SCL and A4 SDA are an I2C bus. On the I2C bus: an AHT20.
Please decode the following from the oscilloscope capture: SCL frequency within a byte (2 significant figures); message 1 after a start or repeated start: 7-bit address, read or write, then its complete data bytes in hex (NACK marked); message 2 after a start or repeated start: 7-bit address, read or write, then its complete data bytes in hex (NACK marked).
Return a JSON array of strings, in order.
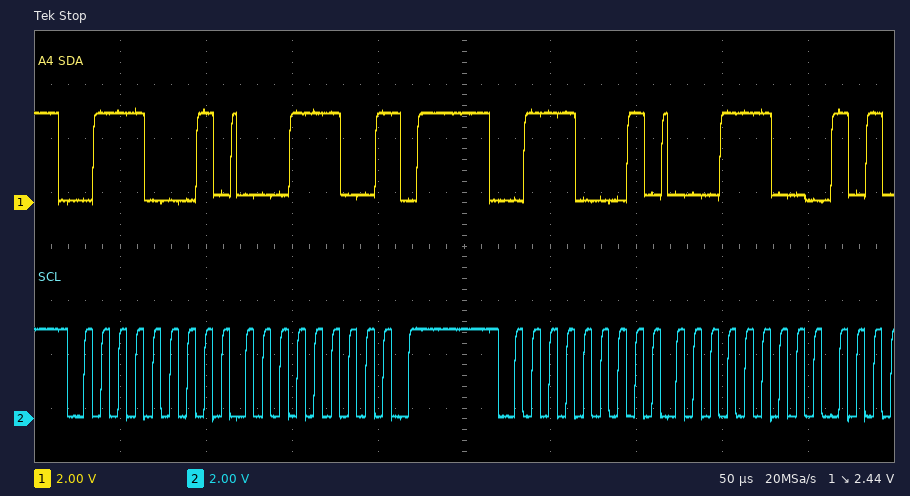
["100 kHz", "0x38 read: 1C NACK", "0x38 read: 1C"]
